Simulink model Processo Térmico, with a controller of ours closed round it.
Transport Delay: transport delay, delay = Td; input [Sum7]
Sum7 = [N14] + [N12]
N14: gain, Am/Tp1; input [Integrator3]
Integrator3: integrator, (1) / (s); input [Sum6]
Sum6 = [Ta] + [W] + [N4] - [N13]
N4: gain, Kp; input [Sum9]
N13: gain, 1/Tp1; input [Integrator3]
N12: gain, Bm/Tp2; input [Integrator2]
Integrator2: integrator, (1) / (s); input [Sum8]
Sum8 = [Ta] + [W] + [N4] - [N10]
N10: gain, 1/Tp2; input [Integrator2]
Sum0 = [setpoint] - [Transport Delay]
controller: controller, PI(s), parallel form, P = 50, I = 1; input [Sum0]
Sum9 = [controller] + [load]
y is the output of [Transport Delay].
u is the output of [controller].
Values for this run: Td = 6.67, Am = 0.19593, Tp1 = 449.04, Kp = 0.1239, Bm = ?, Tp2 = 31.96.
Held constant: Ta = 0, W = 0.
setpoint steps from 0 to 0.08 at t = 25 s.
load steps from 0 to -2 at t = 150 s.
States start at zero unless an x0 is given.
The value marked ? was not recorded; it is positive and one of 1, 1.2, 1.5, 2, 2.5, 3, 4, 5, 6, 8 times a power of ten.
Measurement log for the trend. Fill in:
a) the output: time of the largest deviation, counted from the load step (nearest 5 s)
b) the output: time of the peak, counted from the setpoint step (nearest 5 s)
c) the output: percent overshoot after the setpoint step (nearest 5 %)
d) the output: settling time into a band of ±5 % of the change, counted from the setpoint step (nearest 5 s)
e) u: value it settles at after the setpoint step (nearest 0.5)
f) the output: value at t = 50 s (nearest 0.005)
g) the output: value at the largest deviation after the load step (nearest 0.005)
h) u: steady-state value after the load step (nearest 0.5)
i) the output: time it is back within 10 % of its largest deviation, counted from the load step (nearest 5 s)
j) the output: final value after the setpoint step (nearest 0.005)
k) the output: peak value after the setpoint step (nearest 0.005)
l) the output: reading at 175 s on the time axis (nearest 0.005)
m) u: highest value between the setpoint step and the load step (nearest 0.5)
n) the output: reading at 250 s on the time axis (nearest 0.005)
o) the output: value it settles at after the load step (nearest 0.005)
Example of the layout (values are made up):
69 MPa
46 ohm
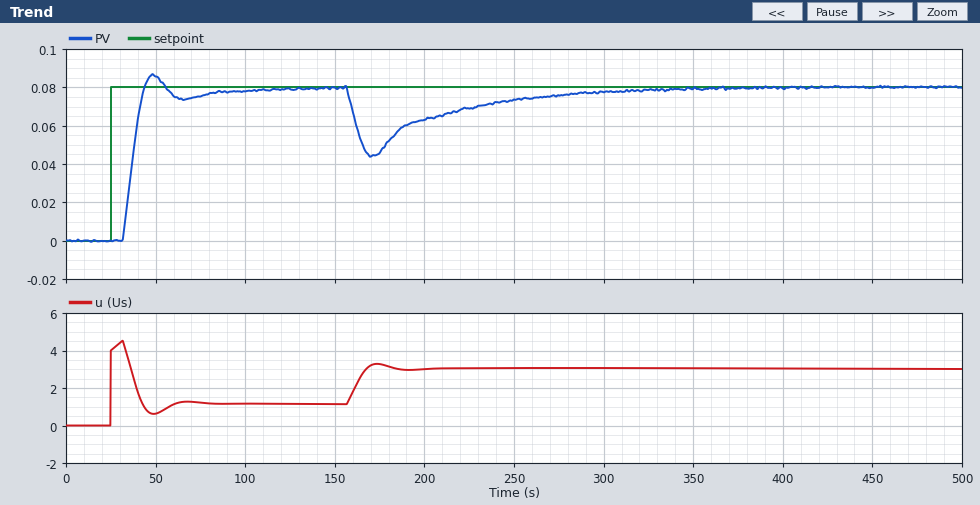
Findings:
20 s
25 s
10 %
50 s
1.0
0.085
0.045
3.0
135 s
0.080
0.085
0.045
4.5
0.075
0.080
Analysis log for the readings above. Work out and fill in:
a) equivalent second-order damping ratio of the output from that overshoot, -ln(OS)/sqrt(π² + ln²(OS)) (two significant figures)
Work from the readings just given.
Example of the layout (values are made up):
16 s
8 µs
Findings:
0.59
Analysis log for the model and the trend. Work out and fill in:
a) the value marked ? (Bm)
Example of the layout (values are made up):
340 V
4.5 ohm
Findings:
0.5
